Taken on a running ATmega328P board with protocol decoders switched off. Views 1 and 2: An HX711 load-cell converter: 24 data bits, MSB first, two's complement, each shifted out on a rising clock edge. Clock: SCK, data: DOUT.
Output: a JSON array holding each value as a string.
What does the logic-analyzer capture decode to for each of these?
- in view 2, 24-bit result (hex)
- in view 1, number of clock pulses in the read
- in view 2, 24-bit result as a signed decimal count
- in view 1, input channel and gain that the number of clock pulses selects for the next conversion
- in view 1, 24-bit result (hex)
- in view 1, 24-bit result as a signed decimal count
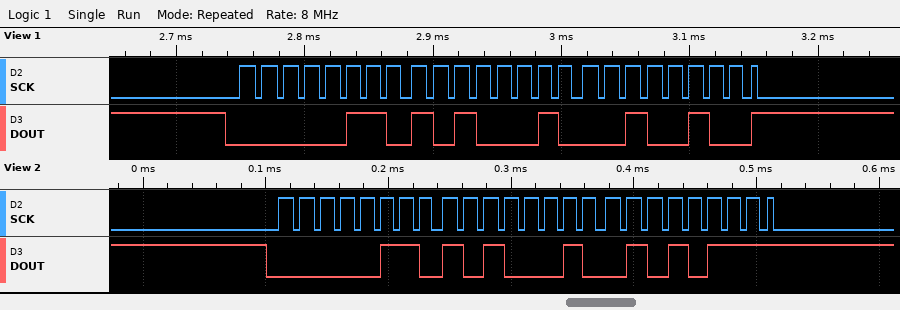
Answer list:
["0x06A257", "25", "434775", "channel A, gain 128", "0x06A224", "434724"]
